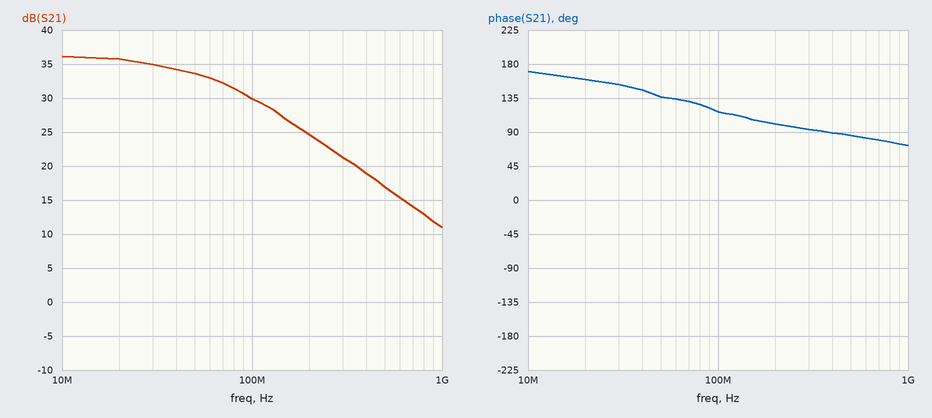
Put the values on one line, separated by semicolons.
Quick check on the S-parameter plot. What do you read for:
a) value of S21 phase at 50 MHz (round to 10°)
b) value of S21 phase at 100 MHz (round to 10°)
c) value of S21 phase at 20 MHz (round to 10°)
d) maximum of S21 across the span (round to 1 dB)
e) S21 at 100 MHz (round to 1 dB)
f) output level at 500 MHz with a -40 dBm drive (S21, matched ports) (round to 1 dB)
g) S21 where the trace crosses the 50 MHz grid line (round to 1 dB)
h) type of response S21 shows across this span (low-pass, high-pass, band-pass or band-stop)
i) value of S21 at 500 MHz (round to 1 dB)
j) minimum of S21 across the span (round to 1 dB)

140°; 120°; 160°; 36 dB; 30 dB; -23 dBm; 34 dB; low-pass; 17 dB; 11 dB
